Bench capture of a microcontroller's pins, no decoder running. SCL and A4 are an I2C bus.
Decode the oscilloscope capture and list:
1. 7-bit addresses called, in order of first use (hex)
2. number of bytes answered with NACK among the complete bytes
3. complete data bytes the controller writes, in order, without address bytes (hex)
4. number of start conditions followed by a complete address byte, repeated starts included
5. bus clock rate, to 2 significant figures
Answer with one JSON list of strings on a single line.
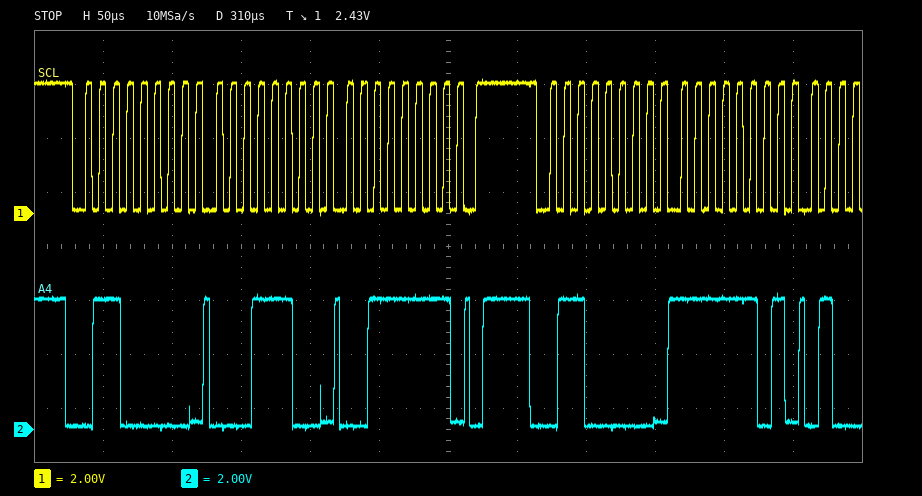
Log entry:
["0x30", "0", "1C 3F FD", "2", "100 kHz"]
